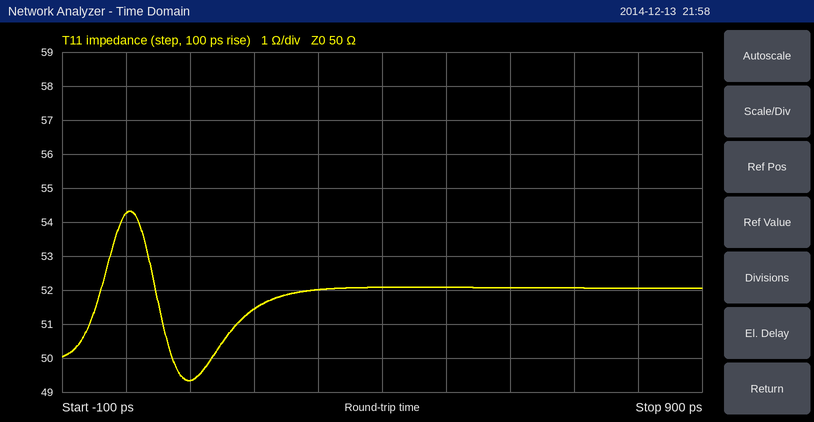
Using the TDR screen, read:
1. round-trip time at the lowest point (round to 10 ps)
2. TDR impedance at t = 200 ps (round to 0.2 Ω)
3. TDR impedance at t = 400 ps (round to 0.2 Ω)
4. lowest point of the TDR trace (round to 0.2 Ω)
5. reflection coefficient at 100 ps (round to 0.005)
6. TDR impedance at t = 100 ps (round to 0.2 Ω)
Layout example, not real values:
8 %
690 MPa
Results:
100 ps
51.4 Ω
52.0 Ω
49.4 Ω
-0.005
49.4 Ω
